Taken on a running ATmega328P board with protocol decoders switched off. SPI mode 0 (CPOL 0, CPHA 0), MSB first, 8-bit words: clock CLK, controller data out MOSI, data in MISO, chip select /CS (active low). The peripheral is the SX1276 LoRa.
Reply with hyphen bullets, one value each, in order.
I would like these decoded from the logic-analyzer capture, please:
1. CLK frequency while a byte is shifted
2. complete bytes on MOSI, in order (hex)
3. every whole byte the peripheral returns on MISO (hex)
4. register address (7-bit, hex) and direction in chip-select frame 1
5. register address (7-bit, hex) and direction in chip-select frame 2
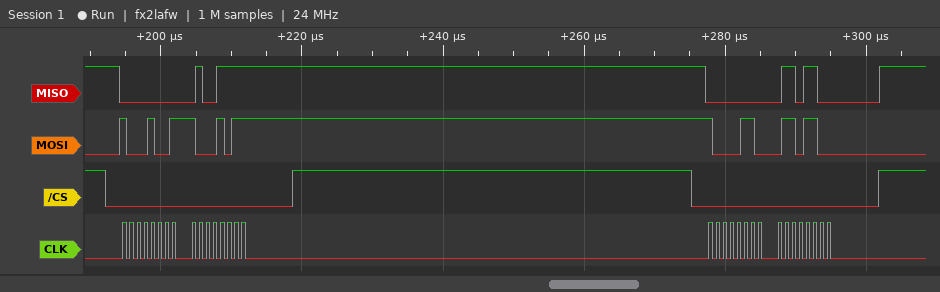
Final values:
- 1 MHz
- 89 8B 86 6C
- 00 4F 00 6C
- 0x09 write
- 0x06 write
